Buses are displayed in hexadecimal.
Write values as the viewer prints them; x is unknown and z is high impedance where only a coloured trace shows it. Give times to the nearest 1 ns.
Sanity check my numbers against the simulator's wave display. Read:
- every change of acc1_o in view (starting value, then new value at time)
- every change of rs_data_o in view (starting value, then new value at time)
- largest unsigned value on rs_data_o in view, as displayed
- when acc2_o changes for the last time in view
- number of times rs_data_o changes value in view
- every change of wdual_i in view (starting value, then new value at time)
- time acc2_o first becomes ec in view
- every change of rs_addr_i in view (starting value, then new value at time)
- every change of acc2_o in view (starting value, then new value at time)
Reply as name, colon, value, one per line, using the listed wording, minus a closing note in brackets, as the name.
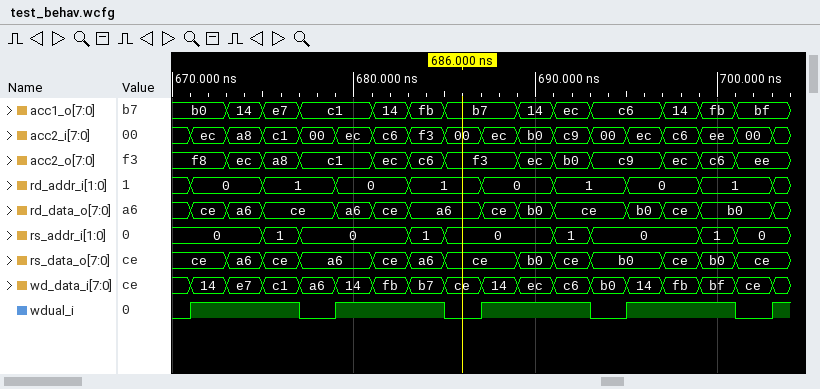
every change of acc1_o in view: b0, 14 at 673 ns, e7 at 675 ns, c1 at 677 ns, 14 at 681 ns, fb at 683 ns, b7 at 685 ns, 14 at 689 ns, ec at 691 ns, c6 at 693 ns, 14 at 697 ns, fb at 699 ns, bf at 701 ns
every change of rs_data_o in view: ce, a6 at 673 ns, ce at 675 ns, a6 at 677 ns, ce at 681 ns, a6 at 683 ns, ce at 685 ns, b0 at 689 ns, ce at 691 ns, b0 at 693 ns, ce at 697 ns, b0 at 699 ns, ce at 701 ns
largest unsigned value on rs_data_o in view, as displayed: ce
when acc2_o changes for the last time in view: 701 ns
number of times rs_data_o changes value in view: 12
every change of wdual_i in view: 0, 1 at 671 ns, 0 at 677 ns, 1 at 679 ns, 0 at 685 ns, 1 at 687 ns, 0 at 693 ns, 1 at 695 ns, 0 at 701 ns, 1 at 703 ns
time acc2_o first becomes ec in view: 673 ns
every change of rs_addr_i in view: 0, 1 at 675 ns, 0 at 677 ns, 1 at 683 ns, 0 at 685 ns, 1 at 691 ns, 0 at 693 ns, 1 at 699 ns, 0 at 701 ns
every change of acc2_o in view: f8, ec at 673 ns, a8 at 675 ns, c1 at 677 ns, ec at 681 ns, c6 at 683 ns, f3 at 685 ns, ec at 689 ns, b0 at 691 ns, c9 at 693 ns, ec at 697 ns, c6 at 699 ns, ee at 701 ns
